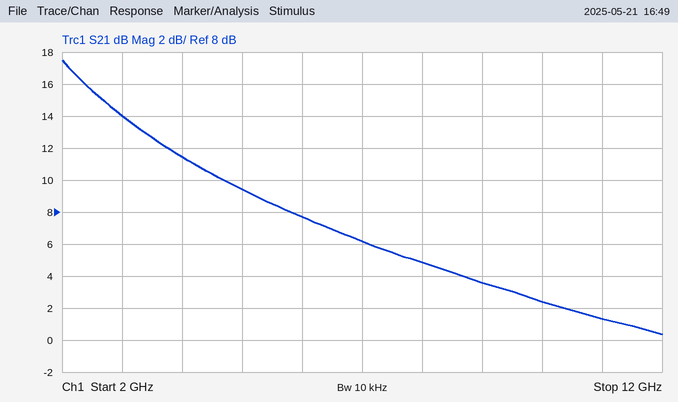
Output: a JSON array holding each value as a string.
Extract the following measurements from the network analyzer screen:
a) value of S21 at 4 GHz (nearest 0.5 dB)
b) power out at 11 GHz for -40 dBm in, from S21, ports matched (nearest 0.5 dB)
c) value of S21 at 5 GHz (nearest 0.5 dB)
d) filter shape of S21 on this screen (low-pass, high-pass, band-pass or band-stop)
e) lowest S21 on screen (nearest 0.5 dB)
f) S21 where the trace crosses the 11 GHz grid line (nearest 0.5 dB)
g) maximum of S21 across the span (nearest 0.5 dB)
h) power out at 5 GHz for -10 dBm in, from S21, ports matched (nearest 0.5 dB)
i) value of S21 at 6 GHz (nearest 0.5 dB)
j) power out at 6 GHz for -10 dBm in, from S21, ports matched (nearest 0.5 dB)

["11.5 dB", "-38.5 dBm", "9.5 dB", "low-pass", "0.5 dB", "1.5 dB", "17.5 dB", "-0.5 dBm", "7.5 dB", "-2.5 dBm"]
